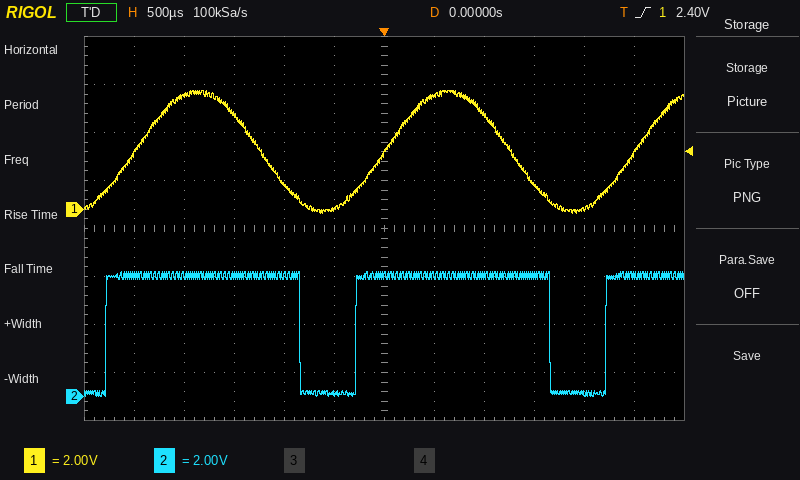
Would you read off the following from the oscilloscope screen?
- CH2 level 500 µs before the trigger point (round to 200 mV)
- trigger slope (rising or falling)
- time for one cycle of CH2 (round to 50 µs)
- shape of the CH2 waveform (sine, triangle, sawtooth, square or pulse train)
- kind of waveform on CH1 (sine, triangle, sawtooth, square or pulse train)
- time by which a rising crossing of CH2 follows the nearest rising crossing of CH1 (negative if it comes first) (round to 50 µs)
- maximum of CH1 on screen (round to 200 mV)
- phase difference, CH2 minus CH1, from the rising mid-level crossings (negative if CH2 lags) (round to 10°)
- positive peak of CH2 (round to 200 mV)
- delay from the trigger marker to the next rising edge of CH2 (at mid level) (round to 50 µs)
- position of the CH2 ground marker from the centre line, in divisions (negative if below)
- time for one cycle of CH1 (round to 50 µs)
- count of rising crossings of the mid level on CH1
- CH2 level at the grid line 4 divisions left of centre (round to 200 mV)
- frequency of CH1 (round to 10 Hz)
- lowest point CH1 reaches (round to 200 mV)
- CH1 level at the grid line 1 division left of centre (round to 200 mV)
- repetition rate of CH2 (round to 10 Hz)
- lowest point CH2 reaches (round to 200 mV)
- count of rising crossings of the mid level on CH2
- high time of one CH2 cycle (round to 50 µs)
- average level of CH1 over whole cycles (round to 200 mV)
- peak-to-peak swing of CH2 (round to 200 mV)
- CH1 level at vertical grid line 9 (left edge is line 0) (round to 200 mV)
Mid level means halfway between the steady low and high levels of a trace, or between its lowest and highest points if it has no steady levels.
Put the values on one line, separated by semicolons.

200 mV; rising; 2.50 ms; pulse train; sine; -300 µs; 5.0 V; +40°; 5.2 V; 2.20 ms; -3.5 div; 2.50 ms; 3; 5.0 V; 400 Hz; -200 mV; 0.0 V; 400 Hz; 0.0 V; 3; 1.95 ms; 2.4 V; 5.2 V; 1.0 V
